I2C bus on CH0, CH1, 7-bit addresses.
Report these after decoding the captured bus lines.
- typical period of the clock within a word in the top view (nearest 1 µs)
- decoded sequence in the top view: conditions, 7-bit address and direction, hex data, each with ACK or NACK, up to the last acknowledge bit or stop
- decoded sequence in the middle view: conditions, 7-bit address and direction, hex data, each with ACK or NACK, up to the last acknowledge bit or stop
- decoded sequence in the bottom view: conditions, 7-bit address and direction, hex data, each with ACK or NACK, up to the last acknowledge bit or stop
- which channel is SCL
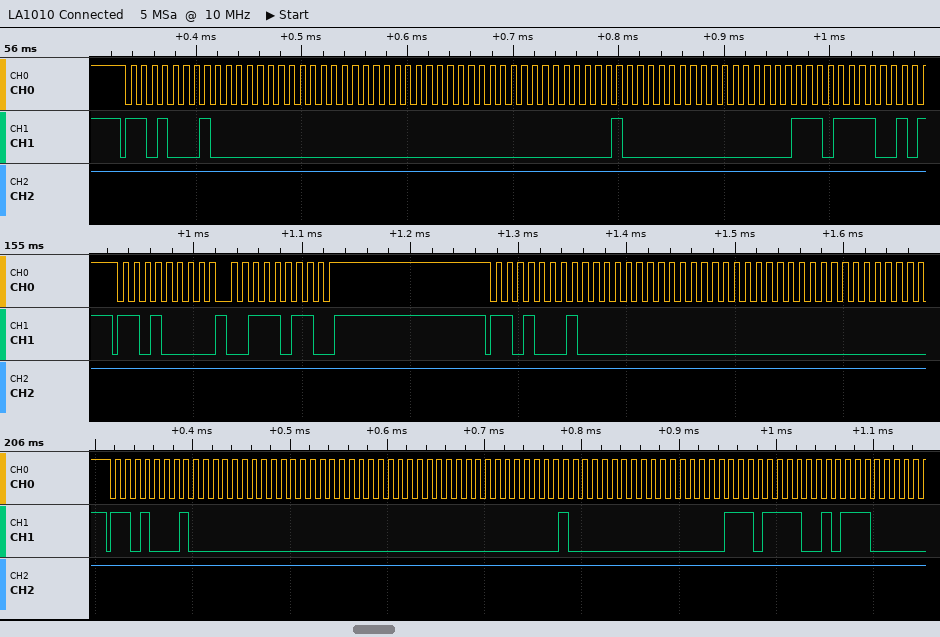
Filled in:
10 µs
start, address 68 read ACK, 00 ACK, 00 ACK, 00 ACK, 00 ACK, 40 ACK, 00 ACK, EF ACK
start, address 68 write ACK, 3B ACK, stop, start, address 68 read ACK, 00 ACK, 00 ACK, 00 ACK
start, address 68 read ACK, 00 ACK, 00 ACK, 00 ACK, 00 ACK, 40 ACK, 00 ACK, EF ACK, 5C ACK
CH0
